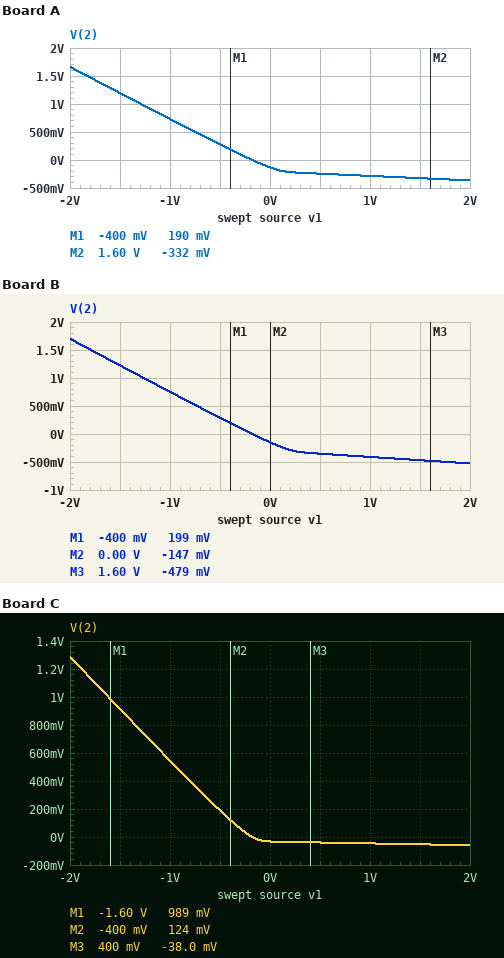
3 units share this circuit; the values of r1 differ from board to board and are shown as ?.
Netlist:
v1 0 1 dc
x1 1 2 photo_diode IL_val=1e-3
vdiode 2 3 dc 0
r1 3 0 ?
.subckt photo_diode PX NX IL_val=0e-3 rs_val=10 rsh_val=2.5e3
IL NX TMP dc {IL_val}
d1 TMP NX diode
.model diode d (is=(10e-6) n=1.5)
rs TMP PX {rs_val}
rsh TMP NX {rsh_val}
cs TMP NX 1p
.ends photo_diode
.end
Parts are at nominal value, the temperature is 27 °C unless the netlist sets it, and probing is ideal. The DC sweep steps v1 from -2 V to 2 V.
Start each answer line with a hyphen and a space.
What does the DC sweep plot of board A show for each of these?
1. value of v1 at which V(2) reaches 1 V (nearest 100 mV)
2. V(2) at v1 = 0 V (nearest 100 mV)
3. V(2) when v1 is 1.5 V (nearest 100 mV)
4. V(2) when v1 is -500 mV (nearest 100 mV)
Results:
- -1.3 V
- -100 mV
- -300 mV
- 300 mV
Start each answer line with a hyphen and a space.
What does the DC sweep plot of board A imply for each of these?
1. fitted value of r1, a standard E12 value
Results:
- 220 Ω
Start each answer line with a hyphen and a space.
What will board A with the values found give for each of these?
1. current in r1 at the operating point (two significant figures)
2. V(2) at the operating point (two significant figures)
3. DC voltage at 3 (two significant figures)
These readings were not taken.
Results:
- 600 µA
- -130 mV
- -130 mV
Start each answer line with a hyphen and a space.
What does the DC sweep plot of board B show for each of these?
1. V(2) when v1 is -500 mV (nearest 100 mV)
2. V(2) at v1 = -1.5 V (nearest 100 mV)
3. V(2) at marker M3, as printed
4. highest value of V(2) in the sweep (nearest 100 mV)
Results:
- 300 mV
- 1.2 V
- -479 mV
- 1.7 V
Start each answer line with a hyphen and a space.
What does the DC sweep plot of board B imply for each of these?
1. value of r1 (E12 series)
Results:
- 330 Ω
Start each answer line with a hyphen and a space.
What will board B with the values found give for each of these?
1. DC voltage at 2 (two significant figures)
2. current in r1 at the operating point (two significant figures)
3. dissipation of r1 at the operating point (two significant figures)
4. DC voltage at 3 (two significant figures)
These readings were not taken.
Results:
- -150 mV
- 450 µA
- 66 µW
- -150 mV
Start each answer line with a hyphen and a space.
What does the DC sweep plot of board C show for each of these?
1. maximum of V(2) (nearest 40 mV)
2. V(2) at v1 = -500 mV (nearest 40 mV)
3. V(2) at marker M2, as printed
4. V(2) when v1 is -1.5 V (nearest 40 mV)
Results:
- 1.28 V
- 200 mV
- 124 mV
- 920 mV
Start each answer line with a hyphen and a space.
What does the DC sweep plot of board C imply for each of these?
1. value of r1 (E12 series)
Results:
- 33 Ω
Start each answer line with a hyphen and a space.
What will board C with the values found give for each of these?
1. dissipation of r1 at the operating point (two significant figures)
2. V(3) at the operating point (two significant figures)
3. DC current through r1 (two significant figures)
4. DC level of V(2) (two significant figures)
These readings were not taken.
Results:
- 31 µW
- -32 mV
- 960 µA
- -32 mV
